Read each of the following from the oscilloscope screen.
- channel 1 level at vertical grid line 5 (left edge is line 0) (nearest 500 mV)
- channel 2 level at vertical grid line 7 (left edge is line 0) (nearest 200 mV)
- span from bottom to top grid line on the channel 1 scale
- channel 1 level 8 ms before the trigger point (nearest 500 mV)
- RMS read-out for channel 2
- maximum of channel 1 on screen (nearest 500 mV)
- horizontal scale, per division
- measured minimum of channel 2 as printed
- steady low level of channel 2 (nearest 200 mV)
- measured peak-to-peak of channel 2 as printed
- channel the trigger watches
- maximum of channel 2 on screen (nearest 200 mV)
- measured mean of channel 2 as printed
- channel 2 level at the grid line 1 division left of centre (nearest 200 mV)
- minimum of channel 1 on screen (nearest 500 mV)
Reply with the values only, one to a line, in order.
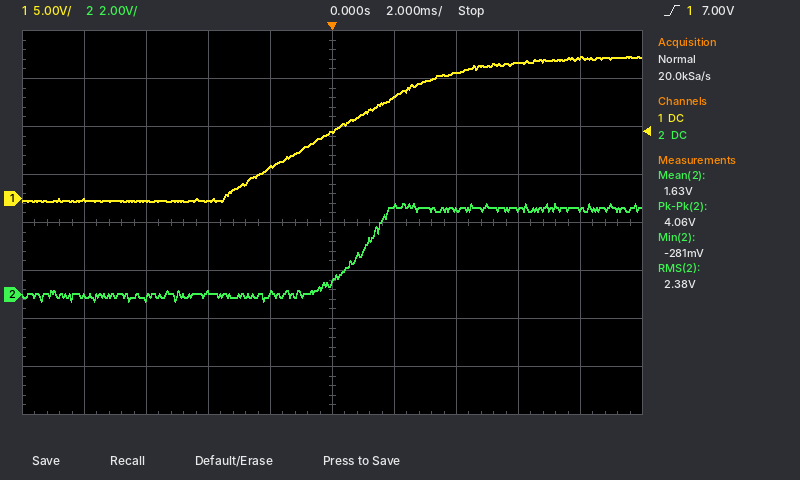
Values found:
7.0 V
3.6 V
40 V
0.0 V
2.38 V
15.0 V
2 ms
-281 mV
0.0 V
4.06 V
channel 1
3.8 V
1.63 V
0.0 V
-500 mV
